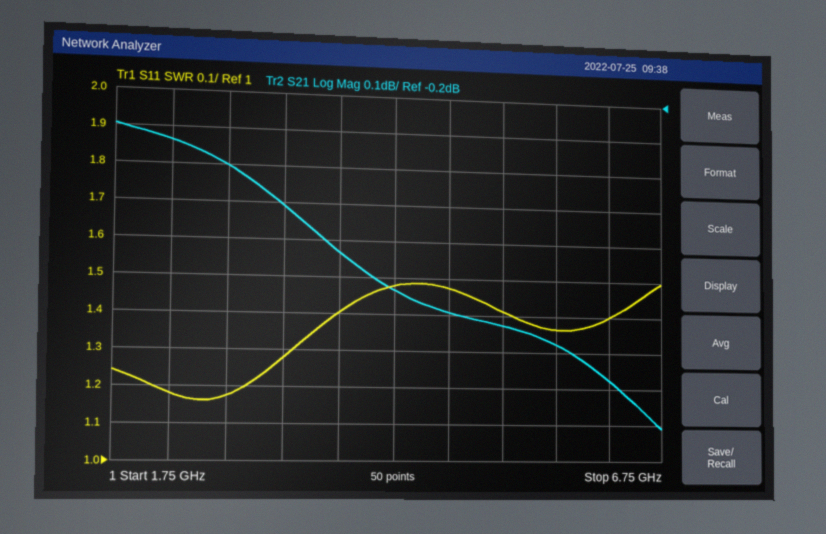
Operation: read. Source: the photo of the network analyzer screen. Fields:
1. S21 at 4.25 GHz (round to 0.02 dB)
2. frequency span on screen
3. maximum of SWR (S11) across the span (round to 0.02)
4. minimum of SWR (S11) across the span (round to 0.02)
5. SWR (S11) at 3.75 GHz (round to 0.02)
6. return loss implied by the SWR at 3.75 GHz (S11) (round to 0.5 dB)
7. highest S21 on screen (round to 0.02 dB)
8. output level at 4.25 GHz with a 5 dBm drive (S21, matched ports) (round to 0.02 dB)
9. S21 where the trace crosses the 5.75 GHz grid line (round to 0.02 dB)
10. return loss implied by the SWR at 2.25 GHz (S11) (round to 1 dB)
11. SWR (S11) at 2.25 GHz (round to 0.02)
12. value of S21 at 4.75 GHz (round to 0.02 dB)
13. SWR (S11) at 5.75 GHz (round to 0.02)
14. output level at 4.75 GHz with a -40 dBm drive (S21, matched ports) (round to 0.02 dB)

-0.74 dB
5 GHz
1.50
1.16
1.40
15.5 dB
-0.30 dB
4.26 dBm
-0.88 dB
22 dB
1.18
-0.80 dB
1.36
-40.80 dBm
